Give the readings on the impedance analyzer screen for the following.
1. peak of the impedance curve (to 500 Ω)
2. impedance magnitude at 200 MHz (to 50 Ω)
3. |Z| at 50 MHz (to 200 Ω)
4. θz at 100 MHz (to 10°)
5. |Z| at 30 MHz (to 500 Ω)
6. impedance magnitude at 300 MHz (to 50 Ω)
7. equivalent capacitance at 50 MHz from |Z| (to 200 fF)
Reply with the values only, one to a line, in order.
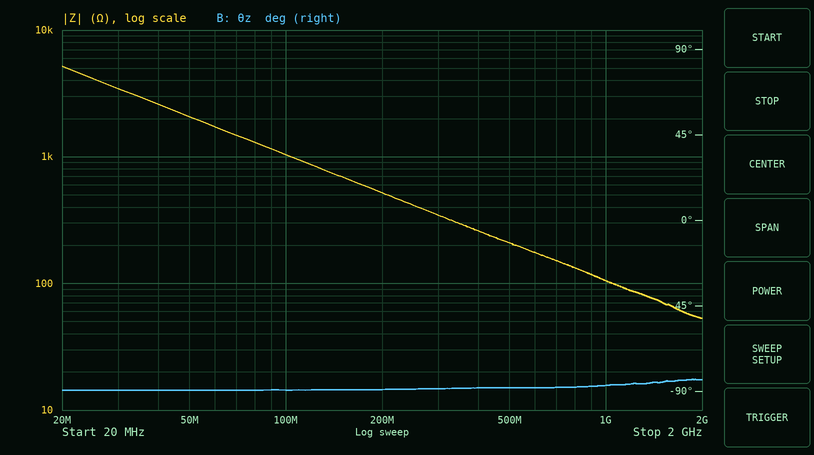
5.0 kΩ
500 Ω
2.0 kΩ
-90°
3.5 kΩ
350 Ω
1.6 pF
